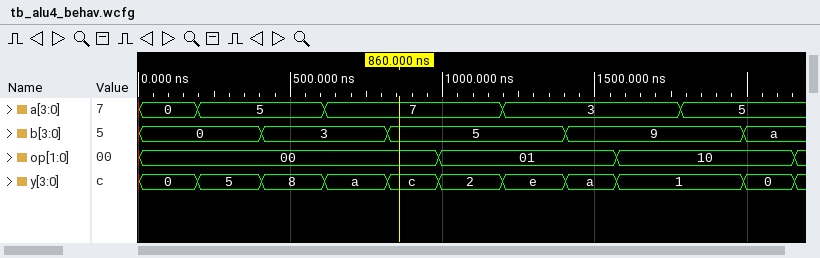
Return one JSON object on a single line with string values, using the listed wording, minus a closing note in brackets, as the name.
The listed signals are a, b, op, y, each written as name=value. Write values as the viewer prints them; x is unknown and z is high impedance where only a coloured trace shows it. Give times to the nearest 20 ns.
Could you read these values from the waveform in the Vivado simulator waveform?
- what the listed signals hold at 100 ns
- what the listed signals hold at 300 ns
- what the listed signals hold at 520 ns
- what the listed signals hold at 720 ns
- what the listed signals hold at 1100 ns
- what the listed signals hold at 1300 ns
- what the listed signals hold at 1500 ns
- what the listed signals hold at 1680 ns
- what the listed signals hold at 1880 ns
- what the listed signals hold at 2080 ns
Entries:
{"what the listed signals hold at 100 ns": "a=0, b=0, op=00, y=0", "what the listed signals hold at 300 ns": "a=5, b=0, op=00, y=5", "what the listed signals hold at 520 ns": "a=5, b=3, op=00, y=8", "what the listed signals hold at 720 ns": "a=7, b=3, op=00, y=a", "what the listed signals hold at 1100 ns": "a=7, b=5, op=01, y=2", "what the listed signals hold at 1300 ns": "a=3, b=5, op=01, y=e", "what the listed signals hold at 1500 ns": "a=3, b=9, op=01, y=a", "what the listed signals hold at 1680 ns": "a=3, b=9, op=10, y=1", "what the listed signals hold at 1880 ns": "a=5, b=9, op=10, y=1", "what the listed signals hold at 2080 ns": "a=5, b=a, op=10, y=0"}
